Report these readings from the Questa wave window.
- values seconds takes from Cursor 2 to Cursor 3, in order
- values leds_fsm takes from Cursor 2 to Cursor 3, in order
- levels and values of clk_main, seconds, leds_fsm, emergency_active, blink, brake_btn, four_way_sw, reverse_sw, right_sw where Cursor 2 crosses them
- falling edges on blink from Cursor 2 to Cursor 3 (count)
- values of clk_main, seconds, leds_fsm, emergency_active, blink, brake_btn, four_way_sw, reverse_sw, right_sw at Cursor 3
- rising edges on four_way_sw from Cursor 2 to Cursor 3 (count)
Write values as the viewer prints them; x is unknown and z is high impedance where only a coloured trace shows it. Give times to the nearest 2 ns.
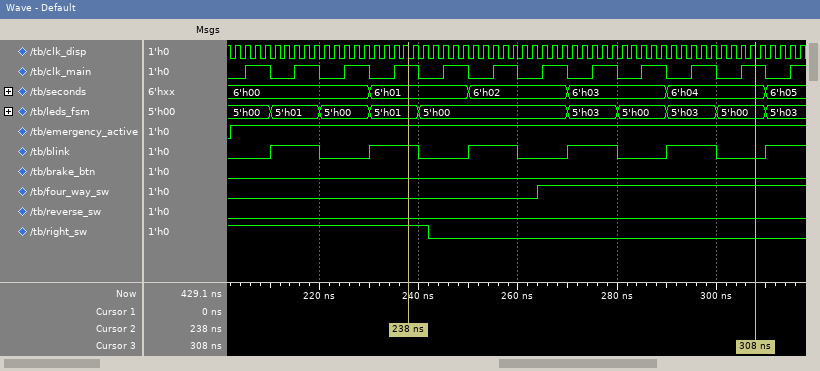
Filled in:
6'h01, 6'h02, 6'h03, 6'h04
5'h01, 5'h00, 5'h03, 5'h00, 5'h03, 5'h00
clk_main=1, seconds=6'h01, leds_fsm=5'h01, emergency_active=1, blink=1, brake_btn=0, four_way_sw=0, reverse_sw=0, right_sw=1
4
clk_main=1, seconds=6'h04, leds_fsm=5'h00, emergency_active=1, blink=0, brake_btn=0, four_way_sw=1, reverse_sw=0, right_sw=0
1
